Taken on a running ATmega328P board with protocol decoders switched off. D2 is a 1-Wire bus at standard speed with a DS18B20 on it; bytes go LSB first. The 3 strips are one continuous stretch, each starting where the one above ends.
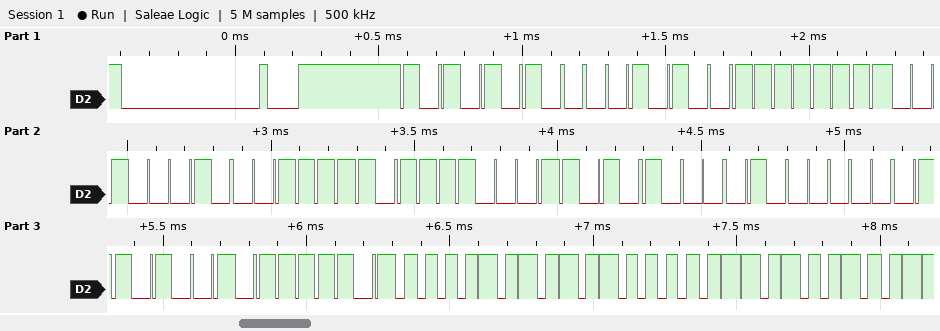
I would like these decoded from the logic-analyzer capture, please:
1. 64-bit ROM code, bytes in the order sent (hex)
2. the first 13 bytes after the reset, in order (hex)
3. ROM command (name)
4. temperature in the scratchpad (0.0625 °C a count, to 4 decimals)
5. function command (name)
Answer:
28 FF 44 7C 8F 15 02 96
55 28 FF 44 7C 8F 15 02 96 BE 50 05 4B
Match ROM
85.0000 °C
Read Scratchpad
